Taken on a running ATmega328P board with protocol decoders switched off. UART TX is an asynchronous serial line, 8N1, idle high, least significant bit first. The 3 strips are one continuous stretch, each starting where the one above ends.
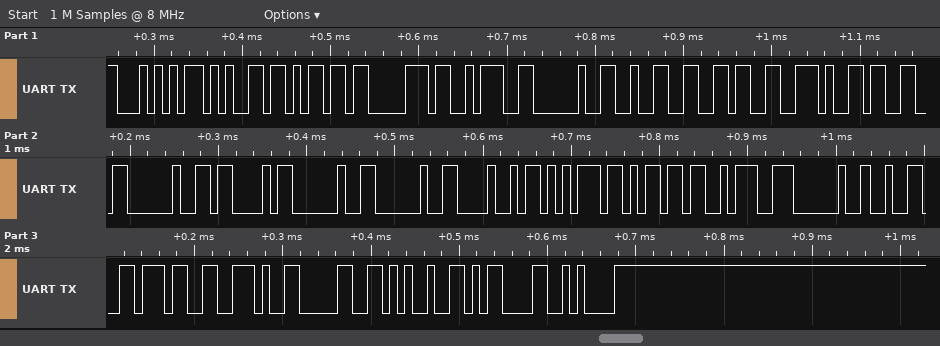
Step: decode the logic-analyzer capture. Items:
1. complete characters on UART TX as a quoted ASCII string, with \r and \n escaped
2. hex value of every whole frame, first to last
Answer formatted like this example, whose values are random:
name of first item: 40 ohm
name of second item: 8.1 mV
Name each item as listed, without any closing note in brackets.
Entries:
complete characters on UART TX as a quoted ASCII string, with \r and \n escaped: "Temp: 26.3 C  Hum: 27.0%\r\n"
hex value of every whole frame, first to last: 54 65 6D 70 3A 20 32 36 2E 33 20 43 20 20 48 75 6D 3A 20 32 37 2E 30 25 0D 0A
